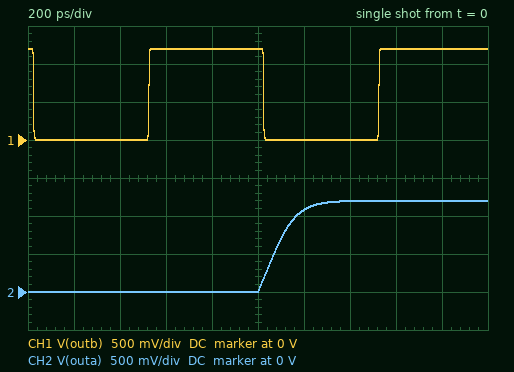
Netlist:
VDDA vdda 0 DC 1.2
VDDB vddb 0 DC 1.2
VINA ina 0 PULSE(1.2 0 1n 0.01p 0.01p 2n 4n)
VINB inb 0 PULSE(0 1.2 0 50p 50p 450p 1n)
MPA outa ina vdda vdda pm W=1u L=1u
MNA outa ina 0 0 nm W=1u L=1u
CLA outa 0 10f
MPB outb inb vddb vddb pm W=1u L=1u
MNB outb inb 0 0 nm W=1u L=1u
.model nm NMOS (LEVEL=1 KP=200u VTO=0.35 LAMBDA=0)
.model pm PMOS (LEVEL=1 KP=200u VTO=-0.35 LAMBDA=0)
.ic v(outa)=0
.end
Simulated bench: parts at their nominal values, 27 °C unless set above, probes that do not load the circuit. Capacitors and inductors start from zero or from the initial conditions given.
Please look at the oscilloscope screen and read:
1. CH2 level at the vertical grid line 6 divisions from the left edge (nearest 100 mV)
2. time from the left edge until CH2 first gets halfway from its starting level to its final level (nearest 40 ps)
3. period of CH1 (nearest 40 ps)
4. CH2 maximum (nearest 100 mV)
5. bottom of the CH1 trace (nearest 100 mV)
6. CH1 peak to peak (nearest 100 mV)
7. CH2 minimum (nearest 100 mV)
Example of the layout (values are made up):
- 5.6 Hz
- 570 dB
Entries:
- 1.1 V
- 1.08 ns
- 1.00 ns
- 1.2 V
- 0 V
- 1.2 V
- 0 V
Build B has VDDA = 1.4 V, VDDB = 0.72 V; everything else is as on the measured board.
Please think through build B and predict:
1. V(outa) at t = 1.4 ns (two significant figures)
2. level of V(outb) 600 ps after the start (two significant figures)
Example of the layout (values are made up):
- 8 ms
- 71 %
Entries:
- 1.4 V
- 720 mV
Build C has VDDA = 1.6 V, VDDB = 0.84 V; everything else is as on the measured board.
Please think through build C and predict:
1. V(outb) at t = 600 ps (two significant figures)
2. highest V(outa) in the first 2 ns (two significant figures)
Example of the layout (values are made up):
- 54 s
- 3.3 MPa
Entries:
- 840 mV
- 1.6 V
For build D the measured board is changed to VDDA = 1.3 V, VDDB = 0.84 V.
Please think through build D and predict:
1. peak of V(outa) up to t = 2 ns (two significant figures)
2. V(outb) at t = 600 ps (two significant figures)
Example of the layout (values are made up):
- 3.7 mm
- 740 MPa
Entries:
- 1.3 V
- 840 mV
